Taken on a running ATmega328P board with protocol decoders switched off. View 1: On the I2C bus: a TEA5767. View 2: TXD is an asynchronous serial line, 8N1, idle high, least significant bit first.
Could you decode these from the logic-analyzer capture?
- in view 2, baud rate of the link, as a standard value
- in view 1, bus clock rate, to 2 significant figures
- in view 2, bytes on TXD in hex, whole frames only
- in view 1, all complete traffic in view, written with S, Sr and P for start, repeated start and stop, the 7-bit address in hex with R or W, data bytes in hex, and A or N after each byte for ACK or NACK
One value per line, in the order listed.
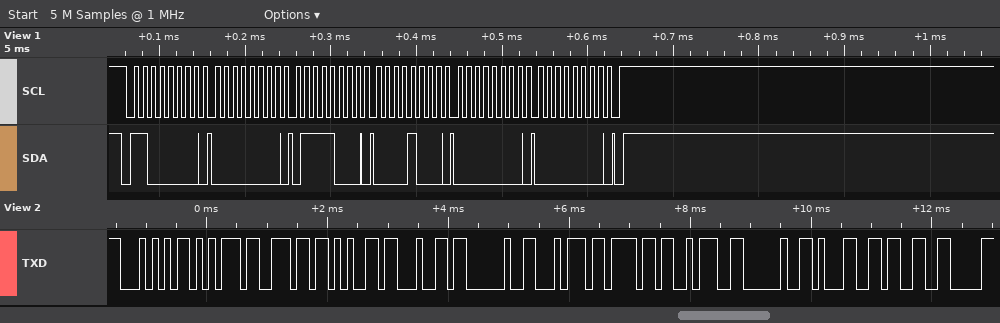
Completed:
9600 baud
100 kHz
0x54 0x75 0x6E 0x65 0x64 0x20 0x74 0x6F 0x3A 0x20 0x31 0x33
S 60W A 00 A 78 A 08 A 00 A 00 A P
